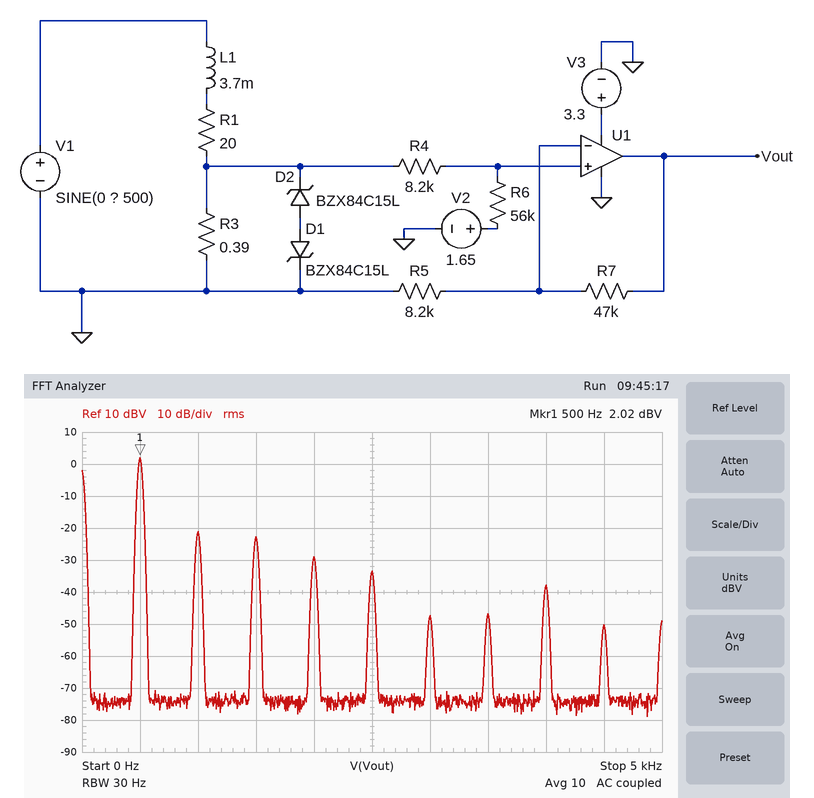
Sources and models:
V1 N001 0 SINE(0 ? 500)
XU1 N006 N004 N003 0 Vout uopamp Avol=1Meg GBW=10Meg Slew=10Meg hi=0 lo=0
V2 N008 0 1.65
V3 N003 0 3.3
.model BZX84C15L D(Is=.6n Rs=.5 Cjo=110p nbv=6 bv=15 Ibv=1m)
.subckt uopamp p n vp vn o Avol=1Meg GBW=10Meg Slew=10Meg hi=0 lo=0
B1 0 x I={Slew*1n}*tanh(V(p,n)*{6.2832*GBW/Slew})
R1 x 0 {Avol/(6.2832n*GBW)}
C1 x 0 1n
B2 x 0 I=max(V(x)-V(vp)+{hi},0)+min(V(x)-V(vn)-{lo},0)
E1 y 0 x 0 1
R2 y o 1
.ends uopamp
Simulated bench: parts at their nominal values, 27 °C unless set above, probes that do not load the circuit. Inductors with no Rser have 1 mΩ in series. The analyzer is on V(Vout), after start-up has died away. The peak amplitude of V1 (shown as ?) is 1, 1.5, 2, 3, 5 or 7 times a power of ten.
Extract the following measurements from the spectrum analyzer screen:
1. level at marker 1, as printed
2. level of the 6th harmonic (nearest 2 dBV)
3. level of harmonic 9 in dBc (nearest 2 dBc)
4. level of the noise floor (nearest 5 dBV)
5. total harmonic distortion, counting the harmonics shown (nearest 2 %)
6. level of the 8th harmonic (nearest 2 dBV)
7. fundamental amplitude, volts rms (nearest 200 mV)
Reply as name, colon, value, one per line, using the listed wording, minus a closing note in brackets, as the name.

level at marker 1, as printed: 2.02 dBV
level of the 6th harmonic: -48 dBV
level of harmonic 9 in dBc: -52 dBc
level of the noise floor: -75 dBV
total harmonic distortion, counting the harmonics shown: 10 %
level of the 8th harmonic: -38 dBV
fundamental amplitude, volts rms: 1.2 V
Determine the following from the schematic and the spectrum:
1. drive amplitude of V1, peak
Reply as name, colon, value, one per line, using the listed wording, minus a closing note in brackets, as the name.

drive amplitude of V1, peak: 20 V
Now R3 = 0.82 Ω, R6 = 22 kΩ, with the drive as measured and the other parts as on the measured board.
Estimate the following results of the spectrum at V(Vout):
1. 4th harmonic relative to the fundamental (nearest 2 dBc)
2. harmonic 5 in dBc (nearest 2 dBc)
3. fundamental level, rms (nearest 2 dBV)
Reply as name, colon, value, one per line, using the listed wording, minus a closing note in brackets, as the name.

4th harmonic relative to the fundamental: -20 dBc
harmonic 5 in dBc: -54 dBc
fundamental level, rms: 2 dBV
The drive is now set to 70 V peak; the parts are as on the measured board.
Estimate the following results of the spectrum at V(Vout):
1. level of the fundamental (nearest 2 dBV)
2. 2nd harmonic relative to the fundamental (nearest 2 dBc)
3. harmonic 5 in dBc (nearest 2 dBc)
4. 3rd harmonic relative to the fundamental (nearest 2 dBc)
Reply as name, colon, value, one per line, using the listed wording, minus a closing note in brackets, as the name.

level of the fundamental: 4 dBV
2nd harmonic relative to the fundamental: -30 dBc
harmonic 5 in dBc: -16 dBc
3rd harmonic relative to the fundamental: -10 dBc
